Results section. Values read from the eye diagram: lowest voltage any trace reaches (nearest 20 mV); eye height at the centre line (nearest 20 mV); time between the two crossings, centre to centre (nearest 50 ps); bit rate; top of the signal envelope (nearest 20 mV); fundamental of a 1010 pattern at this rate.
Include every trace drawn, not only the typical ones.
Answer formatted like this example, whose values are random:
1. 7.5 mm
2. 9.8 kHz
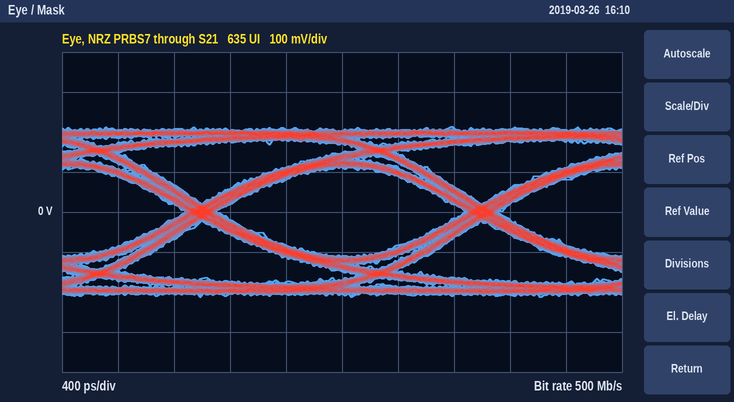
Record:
1. -220 mV
2. 220 mV
3. 2.00 ns
4. 500 Mb/s
5. 220 mV
6. 250 MHz
